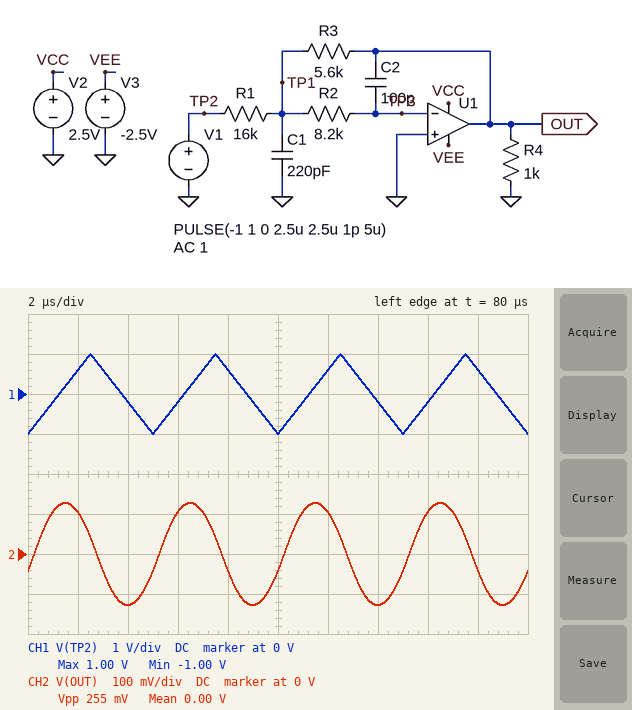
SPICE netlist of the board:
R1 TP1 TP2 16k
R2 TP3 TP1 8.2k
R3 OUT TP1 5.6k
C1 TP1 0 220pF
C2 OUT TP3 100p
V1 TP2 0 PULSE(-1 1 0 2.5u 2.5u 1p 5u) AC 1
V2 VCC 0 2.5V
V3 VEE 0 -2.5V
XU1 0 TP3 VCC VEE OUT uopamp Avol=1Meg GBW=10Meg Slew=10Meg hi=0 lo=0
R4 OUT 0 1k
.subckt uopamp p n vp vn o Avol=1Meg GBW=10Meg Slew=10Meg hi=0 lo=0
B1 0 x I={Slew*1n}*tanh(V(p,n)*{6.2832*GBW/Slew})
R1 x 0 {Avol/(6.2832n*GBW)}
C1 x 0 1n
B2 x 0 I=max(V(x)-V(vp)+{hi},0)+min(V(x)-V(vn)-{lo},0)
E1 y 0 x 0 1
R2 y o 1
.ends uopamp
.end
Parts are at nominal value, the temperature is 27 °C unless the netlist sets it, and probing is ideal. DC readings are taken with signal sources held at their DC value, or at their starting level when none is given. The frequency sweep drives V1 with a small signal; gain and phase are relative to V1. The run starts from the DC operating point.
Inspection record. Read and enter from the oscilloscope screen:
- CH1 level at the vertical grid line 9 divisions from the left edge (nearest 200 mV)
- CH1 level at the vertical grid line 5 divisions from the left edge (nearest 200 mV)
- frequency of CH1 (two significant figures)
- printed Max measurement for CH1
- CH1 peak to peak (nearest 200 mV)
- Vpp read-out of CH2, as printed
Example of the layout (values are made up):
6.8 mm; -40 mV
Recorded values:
600 mV; -1.0 V; 200 kHz; 1.00 V; 2.0 V; 255 mV
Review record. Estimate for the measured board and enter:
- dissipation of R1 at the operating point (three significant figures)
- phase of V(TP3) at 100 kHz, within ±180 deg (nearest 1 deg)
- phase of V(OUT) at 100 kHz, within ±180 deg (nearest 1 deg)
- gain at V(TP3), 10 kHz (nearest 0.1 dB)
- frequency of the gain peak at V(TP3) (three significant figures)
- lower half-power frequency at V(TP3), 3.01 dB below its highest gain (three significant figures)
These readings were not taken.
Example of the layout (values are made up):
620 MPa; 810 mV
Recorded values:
62.5 µW; 29 deg; 119 deg; -69.1 dB; 157 kHz; 74.0 kHz
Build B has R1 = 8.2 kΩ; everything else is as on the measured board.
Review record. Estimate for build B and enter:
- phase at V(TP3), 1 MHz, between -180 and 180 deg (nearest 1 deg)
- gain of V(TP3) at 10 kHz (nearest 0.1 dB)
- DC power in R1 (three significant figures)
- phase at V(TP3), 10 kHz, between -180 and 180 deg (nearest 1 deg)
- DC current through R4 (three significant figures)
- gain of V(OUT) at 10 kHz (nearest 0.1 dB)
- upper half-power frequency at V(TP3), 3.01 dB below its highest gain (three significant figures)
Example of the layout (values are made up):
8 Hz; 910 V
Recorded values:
-78 deg; -63.3 dB; 122 µW; 83 deg; 683 µA; -3.3 dB; 368 kHz
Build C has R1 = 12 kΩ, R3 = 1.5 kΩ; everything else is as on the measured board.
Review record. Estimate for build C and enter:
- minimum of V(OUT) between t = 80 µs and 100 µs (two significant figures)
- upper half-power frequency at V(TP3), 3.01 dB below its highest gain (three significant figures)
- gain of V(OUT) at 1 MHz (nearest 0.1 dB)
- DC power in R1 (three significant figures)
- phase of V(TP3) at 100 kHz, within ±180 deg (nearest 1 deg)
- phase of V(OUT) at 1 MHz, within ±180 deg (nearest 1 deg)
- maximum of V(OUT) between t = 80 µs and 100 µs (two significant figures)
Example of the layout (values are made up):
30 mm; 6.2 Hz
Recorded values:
-70 mV; 741 kHz; -39.7 dB; 83.3 µW; 52 deg; 29 deg; 70 mV
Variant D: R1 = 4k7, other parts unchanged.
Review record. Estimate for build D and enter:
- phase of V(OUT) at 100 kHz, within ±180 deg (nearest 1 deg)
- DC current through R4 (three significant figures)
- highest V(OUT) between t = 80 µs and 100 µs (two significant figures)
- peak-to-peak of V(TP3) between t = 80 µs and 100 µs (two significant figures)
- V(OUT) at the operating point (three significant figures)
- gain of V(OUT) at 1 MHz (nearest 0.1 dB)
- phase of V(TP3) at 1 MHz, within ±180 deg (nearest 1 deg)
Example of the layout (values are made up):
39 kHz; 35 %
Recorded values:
111 deg; 1.19 mA; 310 mV; 14 mV; 1.19 V; -31.1 dB; -75 deg
